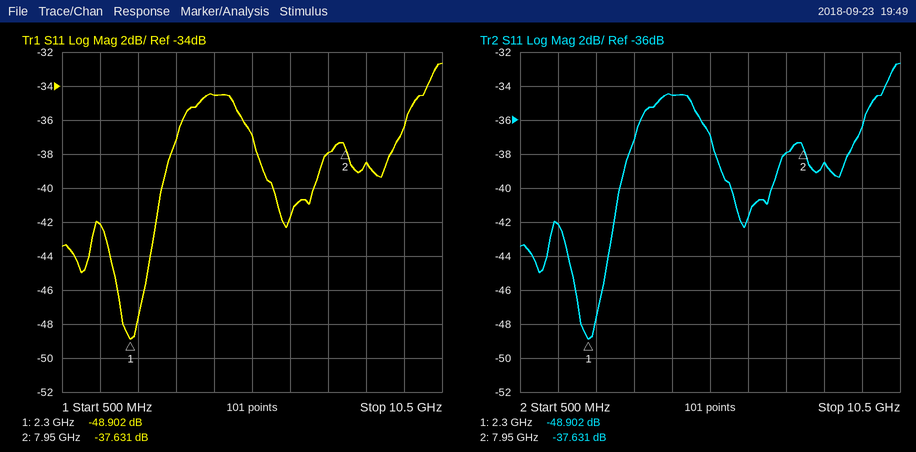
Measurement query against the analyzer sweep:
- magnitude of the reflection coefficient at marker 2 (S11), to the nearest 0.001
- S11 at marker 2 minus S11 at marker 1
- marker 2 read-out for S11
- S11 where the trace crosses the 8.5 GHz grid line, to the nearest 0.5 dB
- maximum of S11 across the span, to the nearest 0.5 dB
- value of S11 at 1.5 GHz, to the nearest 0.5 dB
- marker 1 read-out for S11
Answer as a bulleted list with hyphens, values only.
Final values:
- 0.013
- 11.271 dB
- -37.631 dB
- -38.5 dB
- -32.5 dB
- -42.0 dB
- -48.902 dB
